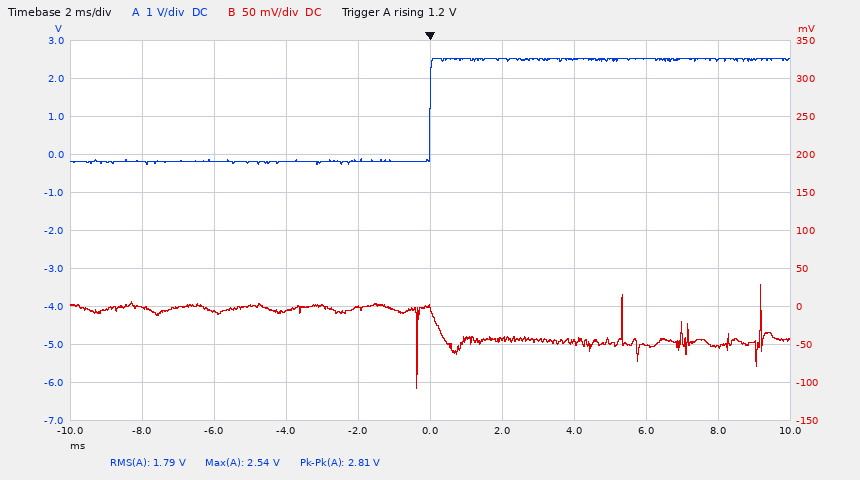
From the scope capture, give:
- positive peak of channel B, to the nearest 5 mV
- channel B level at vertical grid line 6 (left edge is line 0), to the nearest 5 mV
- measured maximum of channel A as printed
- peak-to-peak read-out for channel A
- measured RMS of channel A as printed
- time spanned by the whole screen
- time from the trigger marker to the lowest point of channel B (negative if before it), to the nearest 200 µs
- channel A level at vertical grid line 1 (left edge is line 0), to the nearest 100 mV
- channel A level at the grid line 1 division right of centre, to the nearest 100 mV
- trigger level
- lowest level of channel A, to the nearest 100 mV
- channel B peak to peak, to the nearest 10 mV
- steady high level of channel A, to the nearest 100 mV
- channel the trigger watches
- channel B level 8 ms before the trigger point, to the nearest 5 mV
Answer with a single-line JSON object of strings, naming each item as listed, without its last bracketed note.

{"positive peak of channel B, to the nearest 5 mV": "30 mV", "channel B level at vertical grid line 6 (left edge is line 0), to the nearest 5 mV": "-45 mV", "measured maximum of channel A as printed": "2.54 V", "peak-to-peak read-out for channel A": "2.81 V", "measured RMS of channel A as printed": "1.79 V", "time spanned by the whole screen": "20 ms", "time from the trigger marker to the lowest point of channel B (negative if before it), to the nearest 200 µs": "-400 µs", "channel A level at vertical grid line 1 (left edge is line 0), to the nearest 100 mV": "-200 mV", "channel A level at the grid line 1 division right of centre, to the nearest 100 mV": "2.5 V", "trigger level": "1.2 V", "lowest level of channel A, to the nearest 100 mV": "-300 mV", "channel B peak to peak, to the nearest 10 mV": "140 mV", "steady high level of channel A, to the nearest 100 mV": "2.5 V", "channel the trigger watches": "channel A", "channel B level 8 ms before the trigger point, to the nearest 5 mV": "0 mV"}
